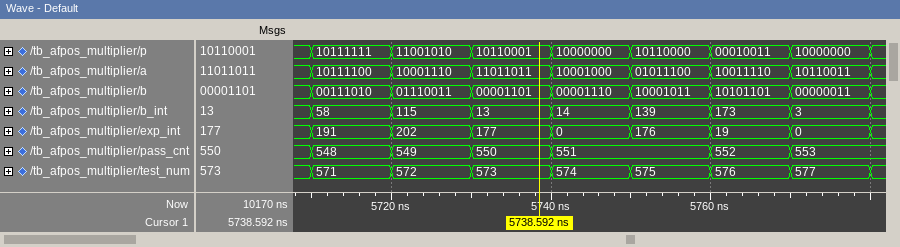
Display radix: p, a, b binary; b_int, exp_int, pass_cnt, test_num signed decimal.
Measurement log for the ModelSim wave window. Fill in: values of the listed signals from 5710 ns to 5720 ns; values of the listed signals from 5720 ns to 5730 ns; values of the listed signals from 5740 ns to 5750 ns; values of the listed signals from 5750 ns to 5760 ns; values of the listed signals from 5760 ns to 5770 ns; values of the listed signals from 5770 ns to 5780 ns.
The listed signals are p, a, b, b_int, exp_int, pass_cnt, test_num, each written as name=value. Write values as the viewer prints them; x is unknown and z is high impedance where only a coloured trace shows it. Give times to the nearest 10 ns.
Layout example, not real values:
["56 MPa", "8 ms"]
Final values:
["p=10111111, a=10111100, b=00111010, b_int=58, exp_int=191, pass_cnt=548, test_num=571", "p=11001010, a=10001110, b=01110011, b_int=115, exp_int=202, pass_cnt=549, test_num=572", "p=10000000, a=10001000, b=00001110, b_int=14, exp_int=0, pass_cnt=551, test_num=574", "p=10110000, a=01011100, b=10001011, b_int=139, exp_int=176, pass_cnt=551, test_num=575", "p=00010011, a=10011110, b=10101101, b_int=173, exp_int=19, pass_cnt=552, test_num=576", "p=10000000, a=10110011, b=00000011, b_int=3, exp_int=0, pass_cnt=553, test_num=577"]
